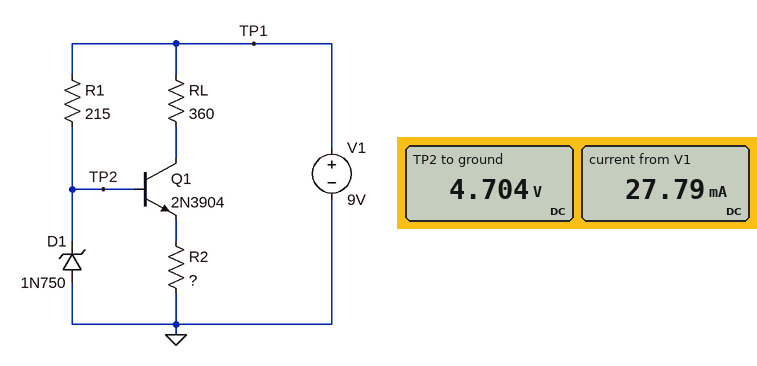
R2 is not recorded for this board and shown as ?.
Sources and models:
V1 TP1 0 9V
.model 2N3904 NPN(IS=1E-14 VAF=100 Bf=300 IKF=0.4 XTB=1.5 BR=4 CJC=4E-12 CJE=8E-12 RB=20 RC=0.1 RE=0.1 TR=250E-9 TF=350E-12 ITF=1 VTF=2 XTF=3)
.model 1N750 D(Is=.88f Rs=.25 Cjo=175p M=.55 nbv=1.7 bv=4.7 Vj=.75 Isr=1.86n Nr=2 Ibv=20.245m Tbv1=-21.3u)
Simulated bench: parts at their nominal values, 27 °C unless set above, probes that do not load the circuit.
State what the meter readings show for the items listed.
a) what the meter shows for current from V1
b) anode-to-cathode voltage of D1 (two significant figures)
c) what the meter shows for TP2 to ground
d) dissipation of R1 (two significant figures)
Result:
27.79 mA
-4.7 V
4.704 V
86 mW
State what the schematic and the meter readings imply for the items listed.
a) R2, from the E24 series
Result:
510 Ω
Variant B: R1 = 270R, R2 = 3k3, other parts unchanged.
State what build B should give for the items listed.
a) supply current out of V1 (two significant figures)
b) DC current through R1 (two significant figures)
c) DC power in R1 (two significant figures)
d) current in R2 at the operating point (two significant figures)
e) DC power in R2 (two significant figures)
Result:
17 mA
16 mA
69 mW
1.2 mA
4.9 mW
